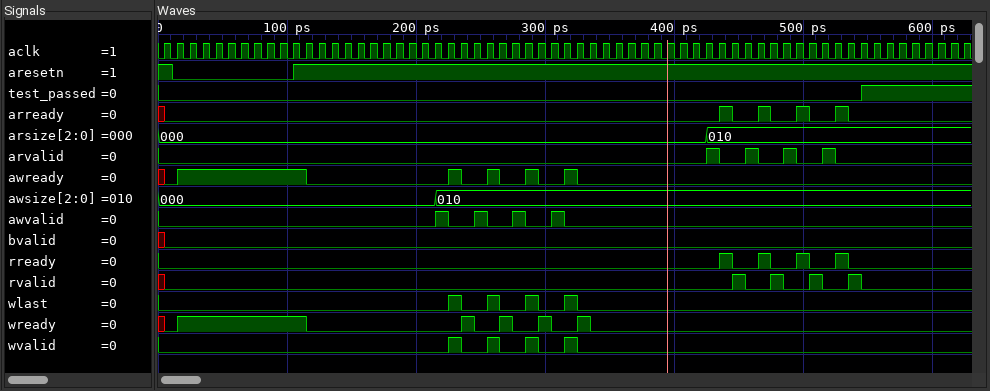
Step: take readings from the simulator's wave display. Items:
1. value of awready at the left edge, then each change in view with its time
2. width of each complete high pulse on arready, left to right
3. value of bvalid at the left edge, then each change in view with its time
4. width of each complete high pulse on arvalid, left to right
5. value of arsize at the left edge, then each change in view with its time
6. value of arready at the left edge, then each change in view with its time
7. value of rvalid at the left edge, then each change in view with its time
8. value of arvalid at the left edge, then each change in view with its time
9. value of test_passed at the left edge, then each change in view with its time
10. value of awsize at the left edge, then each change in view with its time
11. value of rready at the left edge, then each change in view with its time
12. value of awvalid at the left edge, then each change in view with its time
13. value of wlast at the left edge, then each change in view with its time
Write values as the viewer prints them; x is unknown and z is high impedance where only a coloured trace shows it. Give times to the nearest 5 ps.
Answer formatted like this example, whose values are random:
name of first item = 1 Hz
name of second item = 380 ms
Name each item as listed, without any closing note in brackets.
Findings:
value of awready at the left edge, then each change in view with its time = x, 0 at 5 ps, 1 at 15 ps, 0 at 115 ps, 1 at 225 ps, 0 at 235 ps, 1 at 255 ps, 0 at 265 ps, 1 at 285 ps, 0 at 295 ps, 1 at 315 ps, 0 at 325 ps
width of each complete high pulse on arready, left to right = 10 ps, 10 ps, 10 ps, 10 ps
value of bvalid at the left edge, then each change in view with its time = x, 0 at 5 ps
width of each complete high pulse on arvalid, left to right = 10 ps, 10 ps, 10 ps, 10 ps
value of arsize at the left edge, then each change in view with its time = 000, 010 at 425 ps
value of arready at the left edge, then each change in view with its time = x, 0 at 5 ps, 1 at 435 ps, 0 at 445 ps, 1 at 465 ps, 0 at 475 ps, 1 at 495 ps, 0 at 505 ps, 1 at 525 ps, 0 at 535 ps
value of rvalid at the left edge, then each change in view with its time = x, 0 at 5 ps, 1 at 445 ps, 0 at 455 ps, 1 at 475 ps, 0 at 485 ps, 1 at 505 ps, 0 at 515 ps, 1 at 535 ps, 0 at 545 ps
value of arvalid at the left edge, then each change in view with its time = 0, 1 at 425 ps, 0 at 435 ps, 1 at 455 ps, 0 at 465 ps, 1 at 485 ps, 0 at 495 ps, 1 at 515 ps, 0 at 525 ps
value of test_passed at the left edge, then each change in view with its time = 0, 1 at 545 ps
value of awsize at the left edge, then each change in view with its time = 000, 010 at 215 ps
value of rready at the left edge, then each change in view with its time = 0, 1 at 435 ps, 0 at 445 ps, 1 at 465 ps, 0 at 475 ps, 1 at 495 ps, 0 at 505 ps, 1 at 525 ps, 0 at 535 ps
value of awvalid at the left edge, then each change in view with its time = 0, 1 at 215 ps, 0 at 225 ps, 1 at 245 ps, 0 at 255 ps, 1 at 275 ps, 0 at 285 ps, 1 at 305 ps, 0 at 315 ps
value of wlast at the left edge, then each change in view with its time = 0, 1 at 225 ps, 0 at 235 ps, 1 at 255 ps, 0 at 265 ps, 1 at 285 ps, 0 at 295 ps, 1 at 315 ps, 0 at 325 ps
